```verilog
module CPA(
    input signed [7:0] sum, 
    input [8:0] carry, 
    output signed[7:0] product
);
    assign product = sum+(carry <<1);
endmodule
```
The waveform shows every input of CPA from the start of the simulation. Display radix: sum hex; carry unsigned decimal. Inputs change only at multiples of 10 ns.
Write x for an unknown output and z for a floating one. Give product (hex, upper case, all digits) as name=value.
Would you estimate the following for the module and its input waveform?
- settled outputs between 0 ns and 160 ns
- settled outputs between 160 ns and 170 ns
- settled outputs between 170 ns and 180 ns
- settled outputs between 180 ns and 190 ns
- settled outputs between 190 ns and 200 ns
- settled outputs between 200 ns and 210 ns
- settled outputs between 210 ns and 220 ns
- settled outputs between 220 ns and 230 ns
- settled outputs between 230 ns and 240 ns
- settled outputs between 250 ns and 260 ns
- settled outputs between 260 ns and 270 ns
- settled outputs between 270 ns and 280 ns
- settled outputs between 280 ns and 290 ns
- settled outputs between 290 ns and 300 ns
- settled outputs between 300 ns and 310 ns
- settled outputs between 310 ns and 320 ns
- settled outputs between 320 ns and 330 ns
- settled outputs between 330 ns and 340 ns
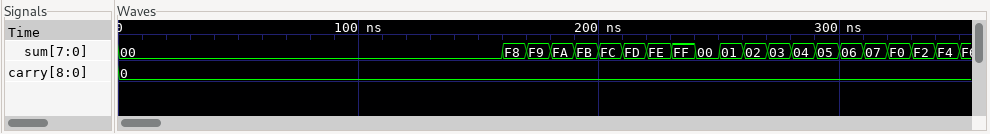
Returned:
product=00
product=F8
product=F9
product=FA
product=FB
product=FC
product=FD
product=FE
product=FF
product=01
product=02
product=03
product=04
product=05
product=06
product=07
product=F0
product=F2
